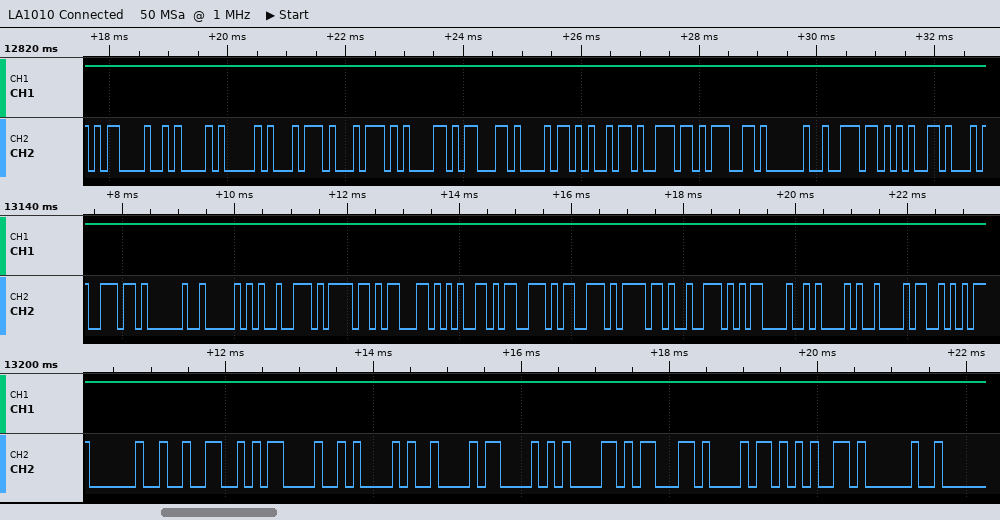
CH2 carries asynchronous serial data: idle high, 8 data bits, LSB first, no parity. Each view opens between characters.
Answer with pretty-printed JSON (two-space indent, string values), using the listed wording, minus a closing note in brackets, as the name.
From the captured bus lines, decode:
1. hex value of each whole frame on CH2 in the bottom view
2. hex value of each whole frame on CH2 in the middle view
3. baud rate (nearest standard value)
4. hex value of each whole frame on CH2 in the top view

{
  "hex value of each whole frame on CH2 in the bottom view": "20, 32, 0D, 0A, 09, 43, 61, 63, 68, 65, 20",
  "hex value of each whole frame on CH2 in the middle view": "6E, 20, 50, 72, 6F, 63, 65, 73, 73, 6F, 72, 0D, 0A, 09, 53",
  "baud rate": "9600 baud",
  "hex value of each whole frame on CH2 in the top view": "0D, 0A, 41, 74, 74, 61, 63, 68, 69, 6E, 67, 20, 6E, 65"
}
